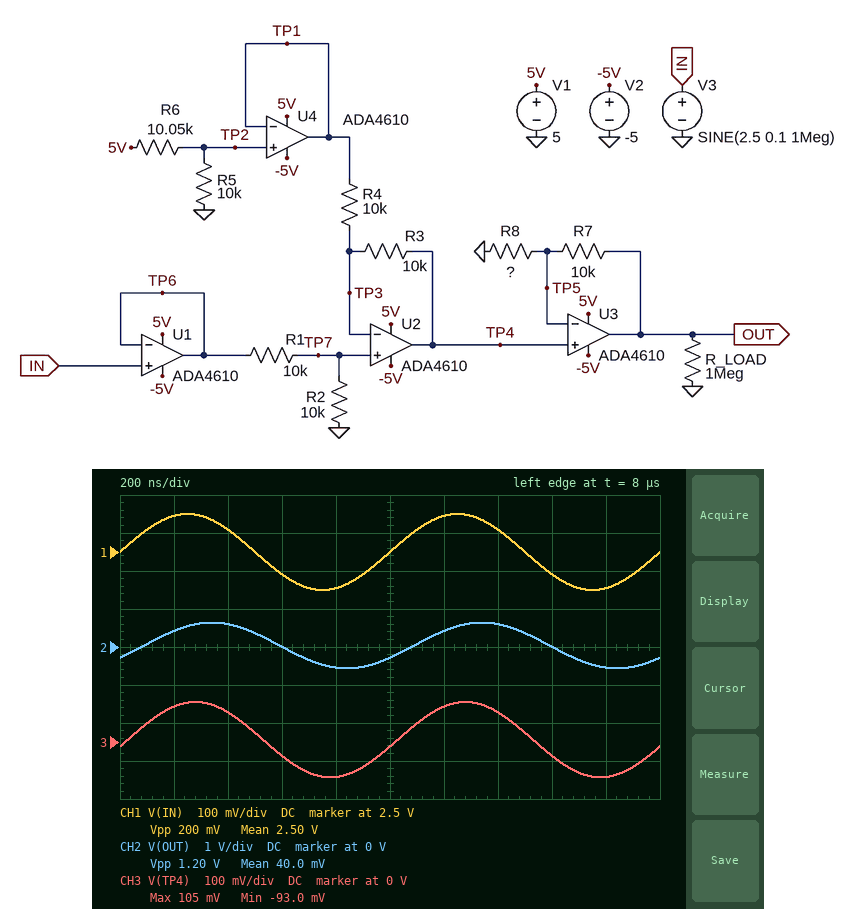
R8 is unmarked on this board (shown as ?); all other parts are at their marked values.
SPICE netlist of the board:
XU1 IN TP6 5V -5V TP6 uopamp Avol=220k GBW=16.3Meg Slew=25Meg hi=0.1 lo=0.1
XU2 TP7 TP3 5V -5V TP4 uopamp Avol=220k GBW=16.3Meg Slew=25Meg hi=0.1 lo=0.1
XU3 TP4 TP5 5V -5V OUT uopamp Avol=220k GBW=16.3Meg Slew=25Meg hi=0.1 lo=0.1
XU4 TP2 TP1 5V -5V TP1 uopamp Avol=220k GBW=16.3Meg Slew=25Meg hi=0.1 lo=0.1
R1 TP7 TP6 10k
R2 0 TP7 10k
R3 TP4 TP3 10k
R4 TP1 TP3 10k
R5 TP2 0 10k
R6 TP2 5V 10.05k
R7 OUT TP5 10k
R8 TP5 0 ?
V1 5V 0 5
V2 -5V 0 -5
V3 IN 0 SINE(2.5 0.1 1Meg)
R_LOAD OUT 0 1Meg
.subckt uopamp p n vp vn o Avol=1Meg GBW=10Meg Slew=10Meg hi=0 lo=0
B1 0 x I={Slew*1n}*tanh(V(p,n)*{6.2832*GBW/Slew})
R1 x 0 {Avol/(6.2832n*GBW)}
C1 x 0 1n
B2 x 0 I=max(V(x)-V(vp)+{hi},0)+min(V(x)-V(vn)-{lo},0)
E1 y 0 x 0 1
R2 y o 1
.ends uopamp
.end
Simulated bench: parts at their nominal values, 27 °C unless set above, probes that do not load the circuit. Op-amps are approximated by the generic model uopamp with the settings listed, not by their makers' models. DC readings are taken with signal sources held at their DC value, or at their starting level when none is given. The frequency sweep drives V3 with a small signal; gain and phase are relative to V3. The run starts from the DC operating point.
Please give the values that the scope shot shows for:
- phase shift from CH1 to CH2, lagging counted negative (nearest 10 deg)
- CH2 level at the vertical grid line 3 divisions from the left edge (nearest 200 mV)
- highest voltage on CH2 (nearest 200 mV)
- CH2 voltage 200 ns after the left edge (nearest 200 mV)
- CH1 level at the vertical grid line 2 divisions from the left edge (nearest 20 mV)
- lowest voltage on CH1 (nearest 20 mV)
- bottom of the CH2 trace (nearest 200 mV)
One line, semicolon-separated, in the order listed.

-30 deg; 0 V; 600 mV; 400 mV; 2.56 V; 2.40 V; -600 mV
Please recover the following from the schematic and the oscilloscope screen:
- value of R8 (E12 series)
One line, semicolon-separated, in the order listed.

1.8 kΩ
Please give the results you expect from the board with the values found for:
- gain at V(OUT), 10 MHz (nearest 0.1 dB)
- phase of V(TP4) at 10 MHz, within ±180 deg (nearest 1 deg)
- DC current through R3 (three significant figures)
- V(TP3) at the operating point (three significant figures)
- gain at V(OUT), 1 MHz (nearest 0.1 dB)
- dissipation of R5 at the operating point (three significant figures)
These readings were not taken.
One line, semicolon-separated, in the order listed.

-1.4 dB; -82 deg; 124 µA; 1.25 V; 15.6 dB; 622 µW
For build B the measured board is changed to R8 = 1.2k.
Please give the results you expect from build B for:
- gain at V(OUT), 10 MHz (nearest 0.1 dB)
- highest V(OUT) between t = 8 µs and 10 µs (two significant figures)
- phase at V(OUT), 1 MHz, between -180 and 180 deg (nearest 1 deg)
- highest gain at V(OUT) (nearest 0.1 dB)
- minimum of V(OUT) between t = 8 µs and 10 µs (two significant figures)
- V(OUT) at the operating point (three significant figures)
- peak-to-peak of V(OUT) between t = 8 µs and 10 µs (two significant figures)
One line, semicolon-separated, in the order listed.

-1.3 dB; 860 mV; -40 deg; 19.4 dB; -740 mV; 58.2 mV; 1.6 V
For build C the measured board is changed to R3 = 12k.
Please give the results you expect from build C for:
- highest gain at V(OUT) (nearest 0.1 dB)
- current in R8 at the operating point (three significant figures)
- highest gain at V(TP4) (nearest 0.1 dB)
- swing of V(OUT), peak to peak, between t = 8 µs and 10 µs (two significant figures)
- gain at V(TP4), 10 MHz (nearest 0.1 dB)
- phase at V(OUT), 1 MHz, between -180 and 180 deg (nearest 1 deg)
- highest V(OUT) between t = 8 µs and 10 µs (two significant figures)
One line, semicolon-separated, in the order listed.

17.2 dB; 135 µA; 0.8 dB; 1.3 V; -5.1 dB; -33 deg; -930 mV
